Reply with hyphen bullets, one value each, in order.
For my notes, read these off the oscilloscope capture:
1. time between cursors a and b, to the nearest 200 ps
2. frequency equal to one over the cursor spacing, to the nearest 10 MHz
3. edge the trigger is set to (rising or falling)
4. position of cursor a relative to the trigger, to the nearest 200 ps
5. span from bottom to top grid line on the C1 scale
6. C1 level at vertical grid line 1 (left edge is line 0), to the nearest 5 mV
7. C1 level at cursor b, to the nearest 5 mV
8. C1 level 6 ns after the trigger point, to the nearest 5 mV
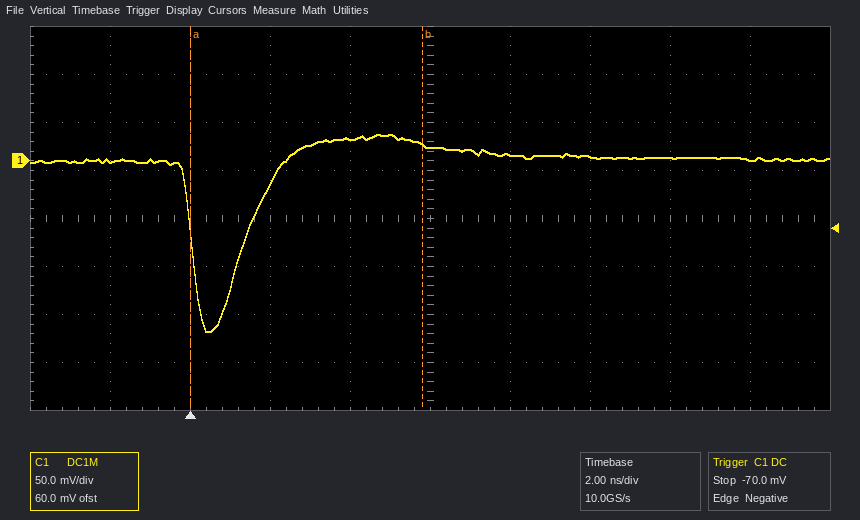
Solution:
- 5.8 ns
- 170 MHz
- falling
- 0.0 ns
- 400 mV
- 0 mV
- 15 mV
- 15 mV
